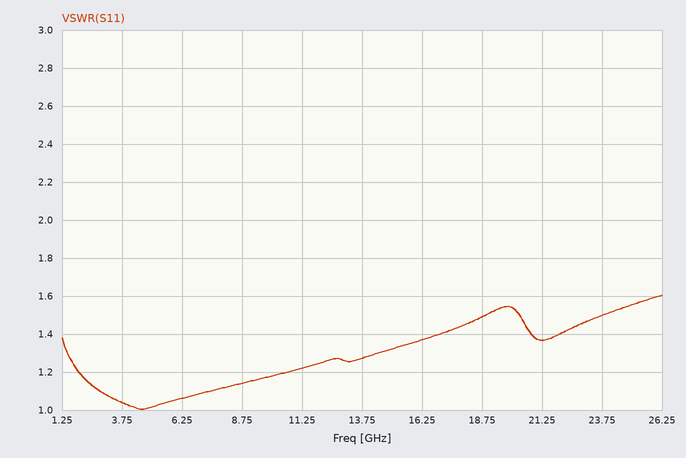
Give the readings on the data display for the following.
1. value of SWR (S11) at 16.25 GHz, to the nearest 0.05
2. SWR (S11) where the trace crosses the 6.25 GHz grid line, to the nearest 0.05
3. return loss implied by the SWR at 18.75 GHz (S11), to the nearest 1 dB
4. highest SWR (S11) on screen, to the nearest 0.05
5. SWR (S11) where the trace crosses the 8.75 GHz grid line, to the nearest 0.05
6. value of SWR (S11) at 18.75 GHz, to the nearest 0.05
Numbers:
1.35
1.05
14 dB
1.60
1.15
1.50
